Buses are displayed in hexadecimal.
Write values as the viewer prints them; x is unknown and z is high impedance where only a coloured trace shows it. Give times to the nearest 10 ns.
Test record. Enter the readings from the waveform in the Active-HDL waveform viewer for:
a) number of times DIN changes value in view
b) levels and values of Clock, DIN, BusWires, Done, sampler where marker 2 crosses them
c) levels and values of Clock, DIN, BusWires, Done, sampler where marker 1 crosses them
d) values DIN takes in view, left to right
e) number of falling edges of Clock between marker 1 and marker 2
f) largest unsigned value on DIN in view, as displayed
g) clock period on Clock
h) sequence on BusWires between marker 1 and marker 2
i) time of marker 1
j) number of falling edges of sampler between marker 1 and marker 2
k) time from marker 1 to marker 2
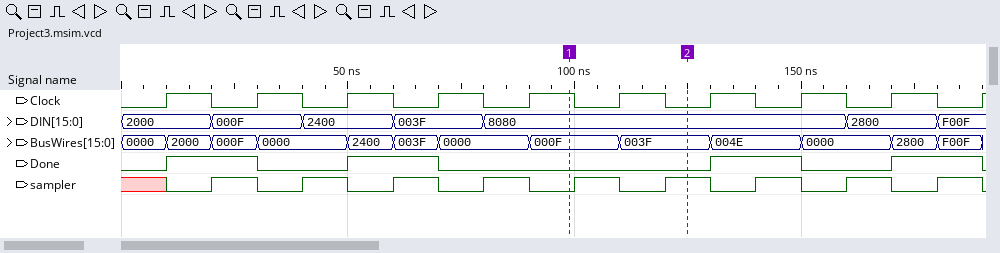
6
Clock=0, DIN=8080, BusWires=003F, Done=0, sampler=1
Clock=1, DIN=8080, BusWires=000F, Done=0, sampler=0
2000, 000F, 2400, 003F, 8080, 2800, F00F
2
F00F
20 ns
000F, 003F
100 ns
1
30 ns
